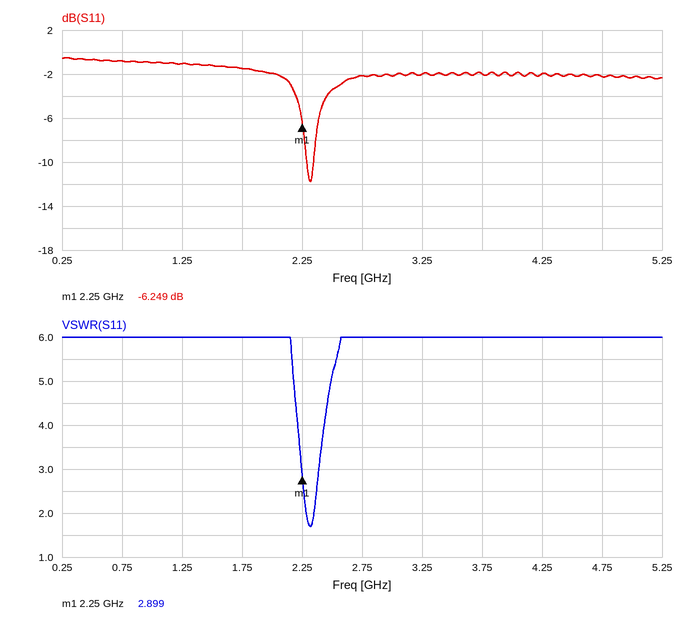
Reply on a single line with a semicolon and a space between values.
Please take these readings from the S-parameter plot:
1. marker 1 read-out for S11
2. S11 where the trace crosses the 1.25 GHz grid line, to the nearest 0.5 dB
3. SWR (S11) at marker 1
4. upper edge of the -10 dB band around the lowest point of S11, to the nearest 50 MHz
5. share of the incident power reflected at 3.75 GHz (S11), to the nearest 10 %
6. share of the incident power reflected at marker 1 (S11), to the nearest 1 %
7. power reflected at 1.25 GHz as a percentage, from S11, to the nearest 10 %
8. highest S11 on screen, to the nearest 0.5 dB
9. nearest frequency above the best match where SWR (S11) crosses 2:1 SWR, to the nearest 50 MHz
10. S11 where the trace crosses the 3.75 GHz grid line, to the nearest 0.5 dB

-6.249 dB; -1.0 dB; 2.899; 2.35 GHz; 60 %; 24 %; 80 %; -0.5 dB; 2.35 GHz; -2.0 dB
